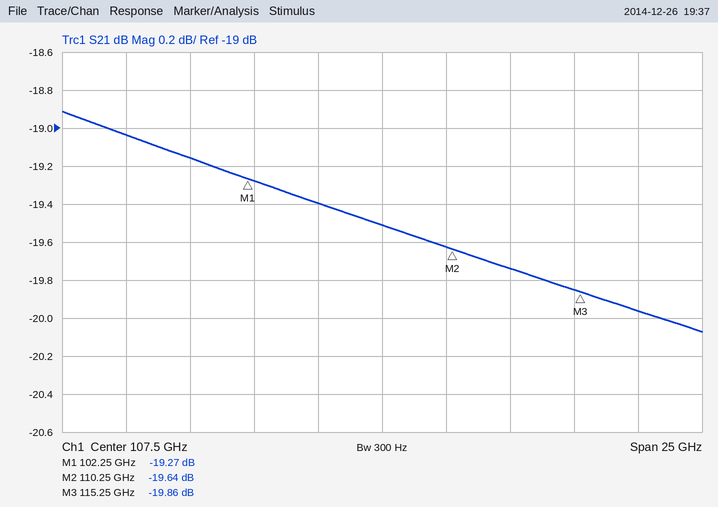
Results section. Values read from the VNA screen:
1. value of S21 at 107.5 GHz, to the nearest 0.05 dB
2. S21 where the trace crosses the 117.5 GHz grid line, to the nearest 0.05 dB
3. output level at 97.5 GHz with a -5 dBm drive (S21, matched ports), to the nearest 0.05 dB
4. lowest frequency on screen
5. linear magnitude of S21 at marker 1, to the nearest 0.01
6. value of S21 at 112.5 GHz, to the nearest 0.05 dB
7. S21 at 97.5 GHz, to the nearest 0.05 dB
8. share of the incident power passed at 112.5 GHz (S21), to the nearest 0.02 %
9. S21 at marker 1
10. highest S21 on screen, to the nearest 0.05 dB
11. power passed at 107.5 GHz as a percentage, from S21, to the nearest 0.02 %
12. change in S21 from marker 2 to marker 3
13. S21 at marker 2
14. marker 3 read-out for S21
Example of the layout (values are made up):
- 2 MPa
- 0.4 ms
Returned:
- -19.50 dB
- -19.95 dB
- -24.05 dBm
- 95 GHz
- 0.11
- -19.75 dB
- -19.05 dB
- 1.06 %
- -19.27 dB
- -18.90 dB
- 1.12 %
- -0.22 dB
- -19.64 dB
- -19.86 dB
